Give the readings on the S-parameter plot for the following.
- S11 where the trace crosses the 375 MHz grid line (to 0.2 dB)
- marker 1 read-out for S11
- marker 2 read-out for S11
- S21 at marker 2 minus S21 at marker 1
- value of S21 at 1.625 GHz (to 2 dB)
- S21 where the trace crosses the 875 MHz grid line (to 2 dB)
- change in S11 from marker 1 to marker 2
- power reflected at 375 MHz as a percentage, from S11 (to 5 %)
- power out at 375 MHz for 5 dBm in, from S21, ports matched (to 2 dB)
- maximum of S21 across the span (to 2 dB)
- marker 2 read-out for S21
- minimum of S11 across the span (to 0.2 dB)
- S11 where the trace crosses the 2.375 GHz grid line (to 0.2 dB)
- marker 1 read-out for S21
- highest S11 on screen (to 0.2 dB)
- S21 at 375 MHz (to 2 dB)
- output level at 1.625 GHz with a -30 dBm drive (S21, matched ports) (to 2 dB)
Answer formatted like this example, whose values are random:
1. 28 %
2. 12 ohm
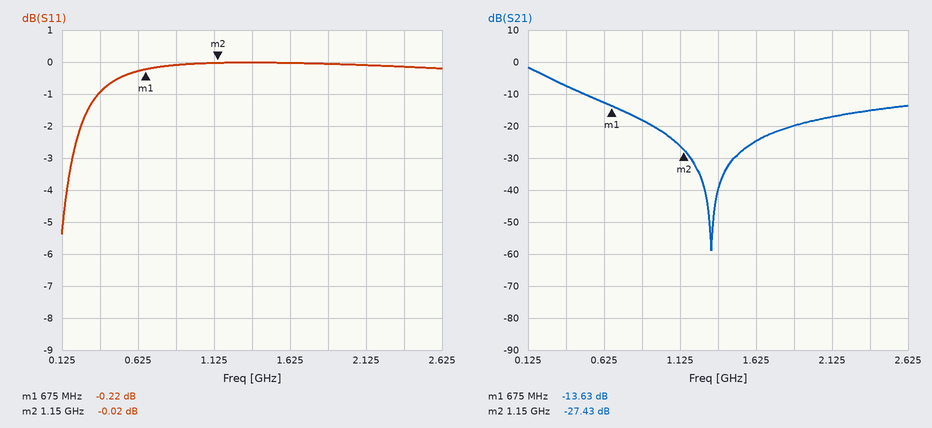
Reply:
1. -1.0 dB
2. -0.22 dB
3. -0.02 dB
4. -13.80 dB
5. -24 dB
6. -18 dB
7. 0.20 dB
8. 80 %
9. -2 dBm
10. -2 dB
11. -27.43 dB
12. -5.4 dB
13. -0.2 dB
14. -13.63 dB
15. 0.0 dB
16. -8 dB
17. -54 dBm
